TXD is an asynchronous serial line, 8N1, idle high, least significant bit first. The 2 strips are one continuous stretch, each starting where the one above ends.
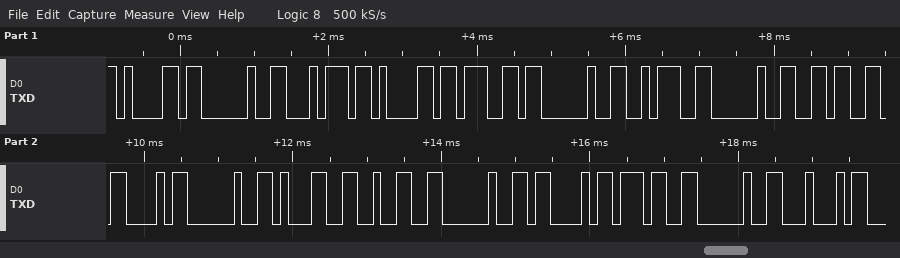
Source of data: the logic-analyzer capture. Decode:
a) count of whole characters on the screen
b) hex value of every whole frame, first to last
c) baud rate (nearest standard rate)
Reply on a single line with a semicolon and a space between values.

18; 61 20 74 61 67 20 3A 20 36 43 20 31 32 20 43 37 20 44; 9600 baud
